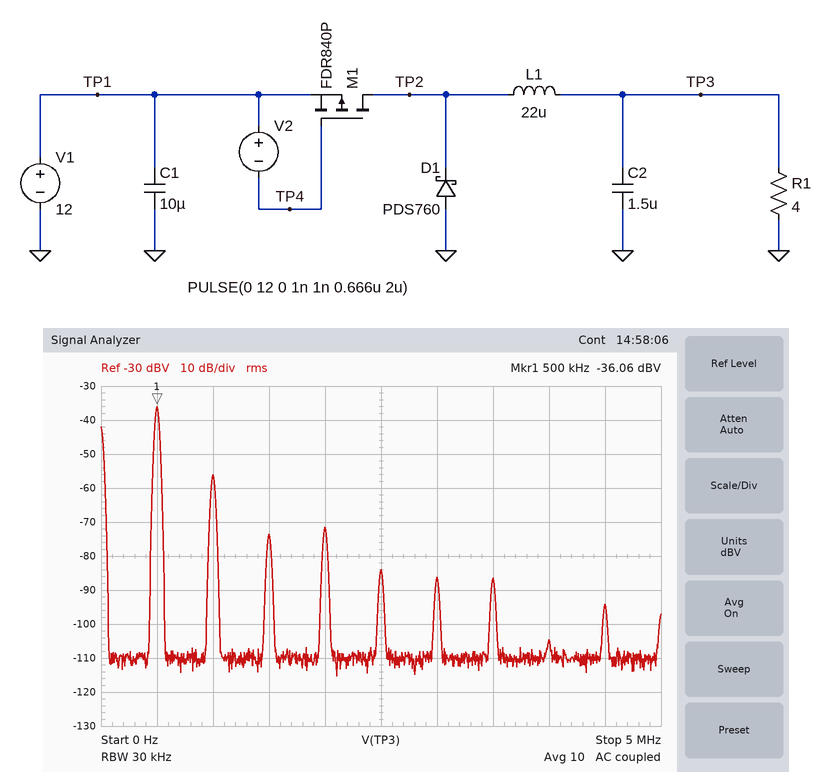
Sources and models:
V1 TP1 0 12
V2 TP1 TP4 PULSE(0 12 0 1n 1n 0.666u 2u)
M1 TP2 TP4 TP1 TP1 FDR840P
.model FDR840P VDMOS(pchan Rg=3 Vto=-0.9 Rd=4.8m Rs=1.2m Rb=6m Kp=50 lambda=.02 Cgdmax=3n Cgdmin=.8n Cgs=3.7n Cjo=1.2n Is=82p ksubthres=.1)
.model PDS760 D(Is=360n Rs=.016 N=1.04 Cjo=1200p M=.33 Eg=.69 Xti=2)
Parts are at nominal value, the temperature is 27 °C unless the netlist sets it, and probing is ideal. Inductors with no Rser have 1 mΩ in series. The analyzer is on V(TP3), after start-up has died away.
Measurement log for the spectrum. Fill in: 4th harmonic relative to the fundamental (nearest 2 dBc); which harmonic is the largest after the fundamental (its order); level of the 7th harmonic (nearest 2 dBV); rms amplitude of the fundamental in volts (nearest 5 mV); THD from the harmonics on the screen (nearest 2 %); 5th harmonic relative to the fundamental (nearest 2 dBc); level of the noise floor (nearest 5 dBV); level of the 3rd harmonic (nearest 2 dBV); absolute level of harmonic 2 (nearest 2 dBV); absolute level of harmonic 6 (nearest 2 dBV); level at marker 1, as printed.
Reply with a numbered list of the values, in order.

1. -36 dBc
2. 2
3. -86 dBV
4. 15 mV
5. 10 %
6. -48 dBc
7. -110 dBV
8. -74 dBV
9. -56 dBV
10. -86 dBV
11. -36.06 dBV
